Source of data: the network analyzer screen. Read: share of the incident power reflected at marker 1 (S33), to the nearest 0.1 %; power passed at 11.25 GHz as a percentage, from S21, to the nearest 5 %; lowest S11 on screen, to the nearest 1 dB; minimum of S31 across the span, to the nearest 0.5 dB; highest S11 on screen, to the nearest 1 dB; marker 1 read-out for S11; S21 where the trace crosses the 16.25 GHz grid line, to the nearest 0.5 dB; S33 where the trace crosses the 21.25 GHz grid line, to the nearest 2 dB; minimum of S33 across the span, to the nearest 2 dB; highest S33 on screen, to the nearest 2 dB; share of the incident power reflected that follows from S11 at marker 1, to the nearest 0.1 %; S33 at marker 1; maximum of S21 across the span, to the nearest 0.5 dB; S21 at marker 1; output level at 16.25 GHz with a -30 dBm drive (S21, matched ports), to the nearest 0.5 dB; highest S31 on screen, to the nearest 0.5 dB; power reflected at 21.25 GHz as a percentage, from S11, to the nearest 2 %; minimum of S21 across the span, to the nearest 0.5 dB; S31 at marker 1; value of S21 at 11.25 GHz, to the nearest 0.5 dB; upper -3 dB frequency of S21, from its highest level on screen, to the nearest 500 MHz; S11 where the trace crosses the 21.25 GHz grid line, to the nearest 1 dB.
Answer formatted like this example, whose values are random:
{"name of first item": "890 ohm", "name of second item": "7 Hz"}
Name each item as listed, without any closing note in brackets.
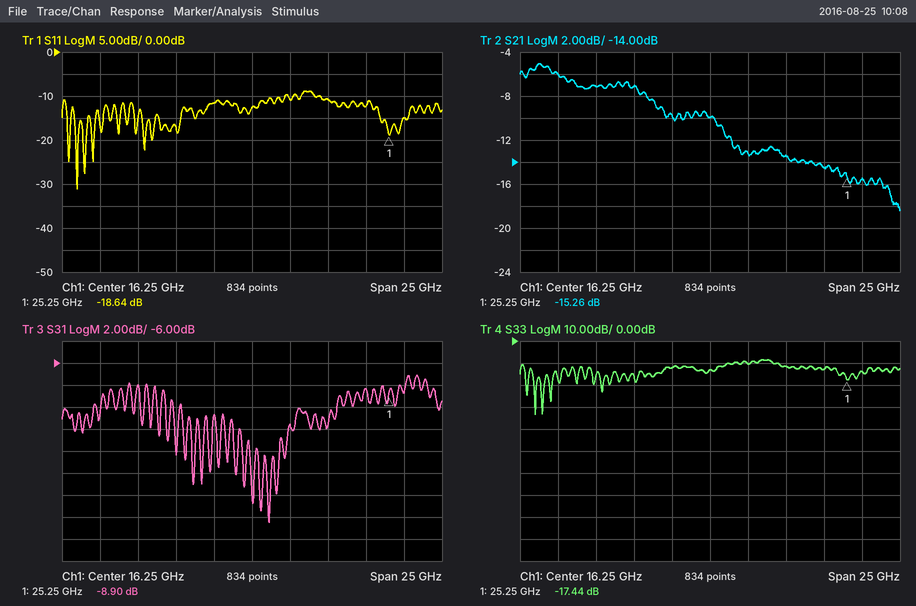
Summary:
{"share of the incident power reflected at marker 1 (S33), to the nearest 0.1 %": "1.8 %", "power passed at 11.25 GHz as a percentage, from S21, to the nearest 5 %": "20 %", "lowest S11 on screen, to the nearest 1 dB": "-31 dB", "minimum of S31 across the span, to the nearest 0.5 dB": "-20.5 dB", "highest S11 on screen, to the nearest 1 dB": "-9 dB", "marker 1 read-out for S11": "-18.64 dB", "S21 where the trace crosses the 16.25 GHz grid line, to the nearest 0.5 dB": "-10.0 dB", "S33 where the trace crosses the 21.25 GHz grid line, to the nearest 2 dB": "-12 dB", "minimum of S33 across the span, to the nearest 2 dB": "-34 dB", "highest S33 on screen, to the nearest 2 dB": "-8 dB", "share of the incident power reflected that follows from S11 at marker 1, to the nearest 0.1 %": "1.4 %", "S33 at marker 1": "-17.44 dB", "maximum of S21 across the span, to the nearest 0.5 dB": "-5.0 dB", "S21 at marker 1": "-15.26 dB", "output level at 16.25 GHz with a -30 dBm drive (S21, matched ports), to the nearest 0.5 dB": "-40.0 dBm", "highest S31 on screen, to the nearest 0.5 dB": "-7.0 dB", "power reflected at 21.25 GHz as a percentage, from S11, to the nearest 2 %": "8 %", "minimum of S21 across the span, to the nearest 0.5 dB": "-18.5 dB", "S31 at marker 1": "-8.90 dB", "value of S21 at 11.25 GHz, to the nearest 0.5 dB": "-7.0 dB", "upper -3 dB frequency of S21, from its highest level on screen, to the nearest 500 MHz": "12.0 GHz", "S11 where the trace crosses the 21.25 GHz grid line, to the nearest 1 dB": "-11 dB"}
